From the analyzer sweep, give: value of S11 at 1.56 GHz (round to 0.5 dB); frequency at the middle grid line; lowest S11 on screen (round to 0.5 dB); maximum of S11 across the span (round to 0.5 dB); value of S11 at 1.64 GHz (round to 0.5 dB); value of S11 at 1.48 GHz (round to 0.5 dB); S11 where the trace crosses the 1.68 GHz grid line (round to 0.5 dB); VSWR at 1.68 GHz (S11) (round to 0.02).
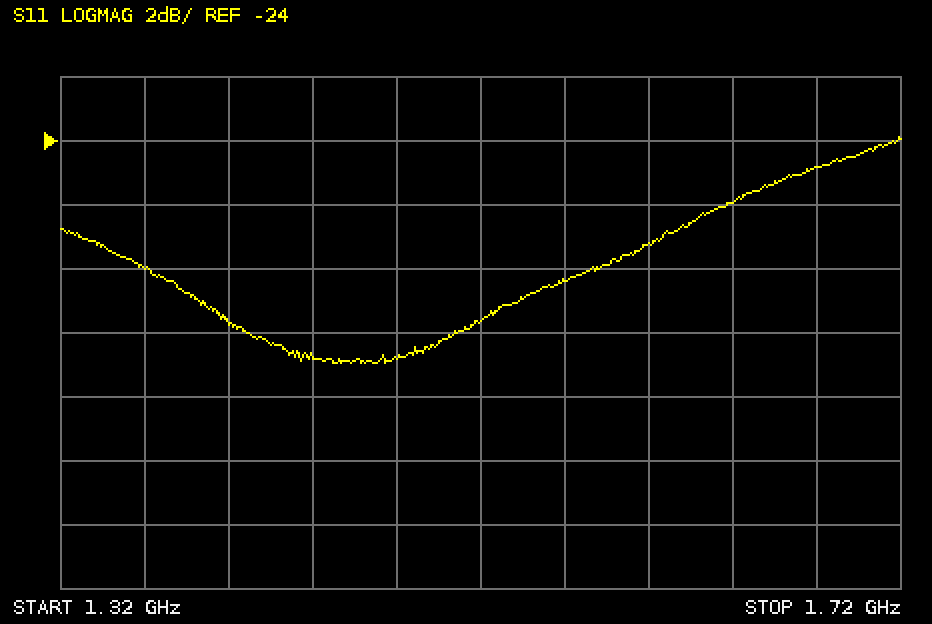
-28.5 dB
1.52 GHz
-31.0 dB
-24.0 dB
-26.0 dB
-31.0 dB
-25.0 dB
1.12
